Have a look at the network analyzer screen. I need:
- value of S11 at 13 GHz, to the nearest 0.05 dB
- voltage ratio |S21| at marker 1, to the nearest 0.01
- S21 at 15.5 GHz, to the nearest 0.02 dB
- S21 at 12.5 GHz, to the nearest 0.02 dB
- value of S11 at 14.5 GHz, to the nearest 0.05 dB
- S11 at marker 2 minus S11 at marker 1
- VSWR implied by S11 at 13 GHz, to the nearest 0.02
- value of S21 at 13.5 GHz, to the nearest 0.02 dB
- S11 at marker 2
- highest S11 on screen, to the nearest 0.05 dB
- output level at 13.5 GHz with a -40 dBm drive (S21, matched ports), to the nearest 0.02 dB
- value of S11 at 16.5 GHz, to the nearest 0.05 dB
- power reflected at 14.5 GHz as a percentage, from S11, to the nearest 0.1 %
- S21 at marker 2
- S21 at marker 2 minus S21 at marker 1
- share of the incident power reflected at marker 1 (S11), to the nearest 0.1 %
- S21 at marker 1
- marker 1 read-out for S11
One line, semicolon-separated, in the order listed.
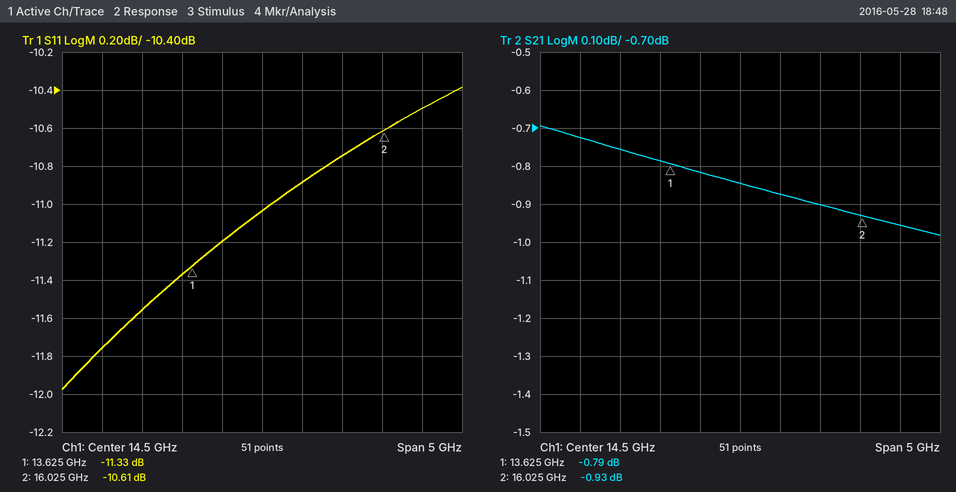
-11.55 dB; 0.91; -0.90 dB; -0.72 dB; -11.05 dB; 0.72 dB; 1.72; -0.78 dB; -10.61 dB; -10.40 dB; -40.78 dBm; -10.50 dB; 7.9 %; -0.93 dB; -0.14 dB; 7.4 %; -0.79 dB; -11.33 dB
